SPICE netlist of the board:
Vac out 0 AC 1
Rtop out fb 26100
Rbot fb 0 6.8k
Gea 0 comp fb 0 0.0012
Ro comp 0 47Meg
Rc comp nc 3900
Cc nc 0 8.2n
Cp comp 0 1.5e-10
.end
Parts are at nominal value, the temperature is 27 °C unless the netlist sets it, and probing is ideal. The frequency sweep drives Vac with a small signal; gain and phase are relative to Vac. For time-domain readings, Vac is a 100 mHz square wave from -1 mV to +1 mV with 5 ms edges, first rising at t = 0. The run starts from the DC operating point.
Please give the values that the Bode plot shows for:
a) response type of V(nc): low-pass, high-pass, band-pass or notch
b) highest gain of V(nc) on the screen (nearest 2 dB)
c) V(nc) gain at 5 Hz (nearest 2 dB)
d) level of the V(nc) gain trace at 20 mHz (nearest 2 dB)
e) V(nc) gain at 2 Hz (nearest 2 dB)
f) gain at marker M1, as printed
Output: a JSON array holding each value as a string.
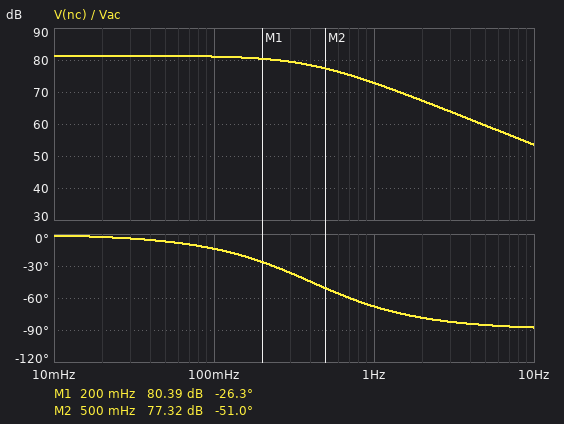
["low-pass", "82 dB", "60 dB", "82 dB", "68 dB", "80.39 dB"]
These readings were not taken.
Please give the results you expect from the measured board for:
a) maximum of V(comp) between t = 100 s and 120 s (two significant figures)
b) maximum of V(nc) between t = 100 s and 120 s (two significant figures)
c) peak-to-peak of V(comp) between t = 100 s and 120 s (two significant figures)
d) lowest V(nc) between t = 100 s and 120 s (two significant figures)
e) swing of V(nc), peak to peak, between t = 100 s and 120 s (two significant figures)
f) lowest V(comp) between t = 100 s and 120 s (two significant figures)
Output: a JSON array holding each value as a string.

["12 V", "12 V", "23 V", "-12 V", "23 V", "-12 V"]
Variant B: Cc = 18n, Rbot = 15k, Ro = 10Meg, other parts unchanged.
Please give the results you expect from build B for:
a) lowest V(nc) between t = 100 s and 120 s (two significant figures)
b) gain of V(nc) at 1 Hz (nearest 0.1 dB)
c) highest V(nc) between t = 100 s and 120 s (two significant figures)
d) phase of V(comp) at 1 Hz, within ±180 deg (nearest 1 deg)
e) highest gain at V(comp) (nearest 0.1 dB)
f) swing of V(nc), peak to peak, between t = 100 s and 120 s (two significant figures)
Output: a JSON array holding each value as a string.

["-4.4 V", "69.2 dB", "4.4 V", "-49 deg", "72.8 dB", "8.8 V"]
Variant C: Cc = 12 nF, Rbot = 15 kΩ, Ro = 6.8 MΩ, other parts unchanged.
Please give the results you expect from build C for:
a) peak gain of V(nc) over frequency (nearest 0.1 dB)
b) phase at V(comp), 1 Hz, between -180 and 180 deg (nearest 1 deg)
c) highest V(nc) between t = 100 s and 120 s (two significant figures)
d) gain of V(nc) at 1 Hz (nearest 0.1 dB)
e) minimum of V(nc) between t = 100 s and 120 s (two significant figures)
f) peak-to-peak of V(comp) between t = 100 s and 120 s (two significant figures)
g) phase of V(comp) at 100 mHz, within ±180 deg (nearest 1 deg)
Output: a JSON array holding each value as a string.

["69.5 dB", "-27 deg", "3.0 V", "68.4 dB", "-3.0 V", "6.0 V", "-3 deg"]
